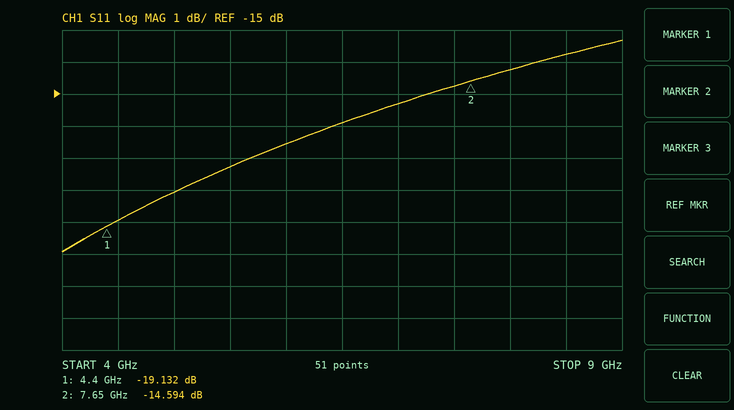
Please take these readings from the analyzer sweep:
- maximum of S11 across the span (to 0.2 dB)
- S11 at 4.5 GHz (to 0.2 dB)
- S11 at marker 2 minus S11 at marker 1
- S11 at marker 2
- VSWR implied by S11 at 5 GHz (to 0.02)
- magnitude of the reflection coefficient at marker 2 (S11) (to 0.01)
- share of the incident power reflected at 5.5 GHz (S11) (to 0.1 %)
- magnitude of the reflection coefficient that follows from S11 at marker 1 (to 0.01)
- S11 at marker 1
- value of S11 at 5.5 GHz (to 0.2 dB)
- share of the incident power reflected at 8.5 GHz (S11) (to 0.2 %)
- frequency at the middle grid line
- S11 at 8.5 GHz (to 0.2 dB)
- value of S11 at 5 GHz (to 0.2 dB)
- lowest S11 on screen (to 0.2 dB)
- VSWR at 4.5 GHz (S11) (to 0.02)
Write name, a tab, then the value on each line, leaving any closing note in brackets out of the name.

maximum of S11 across the span	-13.4 dB
S11 at 4.5 GHz	-19.0 dB
S11 at marker 2 minus S11 at marker 1	4.538 dB
S11 at marker 2	-14.594 dB
VSWR implied by S11 at 5 GHz	1.28
magnitude of the reflection coefficient at marker 2 (S11)	0.19
share of the incident power reflected at 5.5 GHz (S11)	1.9 %
magnitude of the reflection coefficient that follows from S11 at marker 1	0.11
S11 at marker 1	-19.132 dB
value of S11 at 5.5 GHz	-17.2 dB
share of the incident power reflected at 8.5 GHz (S11)	4.2 %
frequency at the middle grid line	6.5 GHz
S11 at 8.5 GHz	-13.8 dB
value of S11 at 5 GHz	-18.0 dB
lowest S11 on screen	-20.0 dB
VSWR at 4.5 GHz (S11)	1.26
